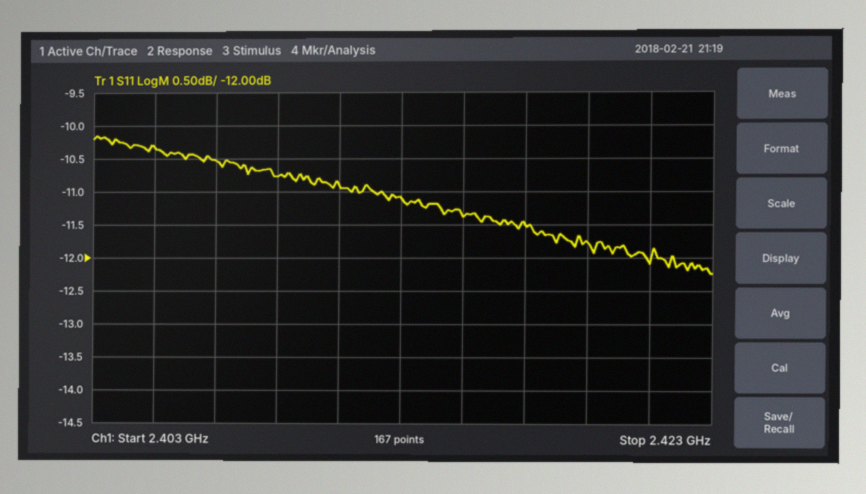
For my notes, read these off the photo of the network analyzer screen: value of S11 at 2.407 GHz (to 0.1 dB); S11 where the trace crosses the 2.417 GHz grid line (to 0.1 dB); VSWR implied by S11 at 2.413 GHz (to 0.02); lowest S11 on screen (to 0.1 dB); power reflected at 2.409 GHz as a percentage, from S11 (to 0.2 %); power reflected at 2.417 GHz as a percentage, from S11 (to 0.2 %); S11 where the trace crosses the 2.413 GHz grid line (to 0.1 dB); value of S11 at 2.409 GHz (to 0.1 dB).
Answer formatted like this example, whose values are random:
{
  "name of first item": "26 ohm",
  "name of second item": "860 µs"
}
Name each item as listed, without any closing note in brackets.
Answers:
{
  "value of S11 at 2.407 GHz": "-10.5 dB",
  "S11 where the trace crosses the 2.417 GHz grid line": "-11.5 dB",
  "VSWR implied by S11 at 2.413 GHz": "1.78",
  "lowest S11 on screen": "-12.2 dB",
  "power reflected at 2.409 GHz as a percentage, from S11": "8.4 %",
  "power reflected at 2.417 GHz as a percentage, from S11": "7.0 %",
  "S11 where the trace crosses the 2.413 GHz grid line": "-11.1 dB",
  "value of S11 at 2.409 GHz": "-10.8 dB"
}
